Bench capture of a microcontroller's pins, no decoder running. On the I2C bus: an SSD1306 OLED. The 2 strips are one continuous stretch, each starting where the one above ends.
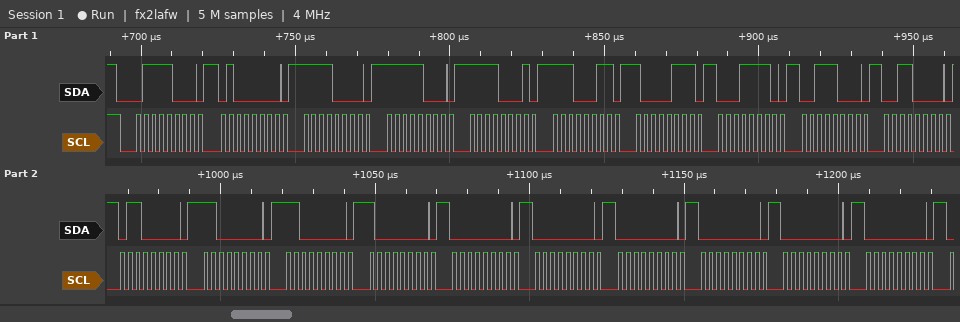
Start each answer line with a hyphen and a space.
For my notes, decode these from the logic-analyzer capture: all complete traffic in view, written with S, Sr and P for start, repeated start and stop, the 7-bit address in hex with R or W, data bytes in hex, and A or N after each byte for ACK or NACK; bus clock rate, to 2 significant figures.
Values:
- S 3CW A 40 A F0 A F8 A F1 A E3 A 87 A 1E A 38 A 30 A 60 A C0 A C0 A 80 A 00 A 00 A 00 A 00 A 00 A 00 A
- 400 kHz
